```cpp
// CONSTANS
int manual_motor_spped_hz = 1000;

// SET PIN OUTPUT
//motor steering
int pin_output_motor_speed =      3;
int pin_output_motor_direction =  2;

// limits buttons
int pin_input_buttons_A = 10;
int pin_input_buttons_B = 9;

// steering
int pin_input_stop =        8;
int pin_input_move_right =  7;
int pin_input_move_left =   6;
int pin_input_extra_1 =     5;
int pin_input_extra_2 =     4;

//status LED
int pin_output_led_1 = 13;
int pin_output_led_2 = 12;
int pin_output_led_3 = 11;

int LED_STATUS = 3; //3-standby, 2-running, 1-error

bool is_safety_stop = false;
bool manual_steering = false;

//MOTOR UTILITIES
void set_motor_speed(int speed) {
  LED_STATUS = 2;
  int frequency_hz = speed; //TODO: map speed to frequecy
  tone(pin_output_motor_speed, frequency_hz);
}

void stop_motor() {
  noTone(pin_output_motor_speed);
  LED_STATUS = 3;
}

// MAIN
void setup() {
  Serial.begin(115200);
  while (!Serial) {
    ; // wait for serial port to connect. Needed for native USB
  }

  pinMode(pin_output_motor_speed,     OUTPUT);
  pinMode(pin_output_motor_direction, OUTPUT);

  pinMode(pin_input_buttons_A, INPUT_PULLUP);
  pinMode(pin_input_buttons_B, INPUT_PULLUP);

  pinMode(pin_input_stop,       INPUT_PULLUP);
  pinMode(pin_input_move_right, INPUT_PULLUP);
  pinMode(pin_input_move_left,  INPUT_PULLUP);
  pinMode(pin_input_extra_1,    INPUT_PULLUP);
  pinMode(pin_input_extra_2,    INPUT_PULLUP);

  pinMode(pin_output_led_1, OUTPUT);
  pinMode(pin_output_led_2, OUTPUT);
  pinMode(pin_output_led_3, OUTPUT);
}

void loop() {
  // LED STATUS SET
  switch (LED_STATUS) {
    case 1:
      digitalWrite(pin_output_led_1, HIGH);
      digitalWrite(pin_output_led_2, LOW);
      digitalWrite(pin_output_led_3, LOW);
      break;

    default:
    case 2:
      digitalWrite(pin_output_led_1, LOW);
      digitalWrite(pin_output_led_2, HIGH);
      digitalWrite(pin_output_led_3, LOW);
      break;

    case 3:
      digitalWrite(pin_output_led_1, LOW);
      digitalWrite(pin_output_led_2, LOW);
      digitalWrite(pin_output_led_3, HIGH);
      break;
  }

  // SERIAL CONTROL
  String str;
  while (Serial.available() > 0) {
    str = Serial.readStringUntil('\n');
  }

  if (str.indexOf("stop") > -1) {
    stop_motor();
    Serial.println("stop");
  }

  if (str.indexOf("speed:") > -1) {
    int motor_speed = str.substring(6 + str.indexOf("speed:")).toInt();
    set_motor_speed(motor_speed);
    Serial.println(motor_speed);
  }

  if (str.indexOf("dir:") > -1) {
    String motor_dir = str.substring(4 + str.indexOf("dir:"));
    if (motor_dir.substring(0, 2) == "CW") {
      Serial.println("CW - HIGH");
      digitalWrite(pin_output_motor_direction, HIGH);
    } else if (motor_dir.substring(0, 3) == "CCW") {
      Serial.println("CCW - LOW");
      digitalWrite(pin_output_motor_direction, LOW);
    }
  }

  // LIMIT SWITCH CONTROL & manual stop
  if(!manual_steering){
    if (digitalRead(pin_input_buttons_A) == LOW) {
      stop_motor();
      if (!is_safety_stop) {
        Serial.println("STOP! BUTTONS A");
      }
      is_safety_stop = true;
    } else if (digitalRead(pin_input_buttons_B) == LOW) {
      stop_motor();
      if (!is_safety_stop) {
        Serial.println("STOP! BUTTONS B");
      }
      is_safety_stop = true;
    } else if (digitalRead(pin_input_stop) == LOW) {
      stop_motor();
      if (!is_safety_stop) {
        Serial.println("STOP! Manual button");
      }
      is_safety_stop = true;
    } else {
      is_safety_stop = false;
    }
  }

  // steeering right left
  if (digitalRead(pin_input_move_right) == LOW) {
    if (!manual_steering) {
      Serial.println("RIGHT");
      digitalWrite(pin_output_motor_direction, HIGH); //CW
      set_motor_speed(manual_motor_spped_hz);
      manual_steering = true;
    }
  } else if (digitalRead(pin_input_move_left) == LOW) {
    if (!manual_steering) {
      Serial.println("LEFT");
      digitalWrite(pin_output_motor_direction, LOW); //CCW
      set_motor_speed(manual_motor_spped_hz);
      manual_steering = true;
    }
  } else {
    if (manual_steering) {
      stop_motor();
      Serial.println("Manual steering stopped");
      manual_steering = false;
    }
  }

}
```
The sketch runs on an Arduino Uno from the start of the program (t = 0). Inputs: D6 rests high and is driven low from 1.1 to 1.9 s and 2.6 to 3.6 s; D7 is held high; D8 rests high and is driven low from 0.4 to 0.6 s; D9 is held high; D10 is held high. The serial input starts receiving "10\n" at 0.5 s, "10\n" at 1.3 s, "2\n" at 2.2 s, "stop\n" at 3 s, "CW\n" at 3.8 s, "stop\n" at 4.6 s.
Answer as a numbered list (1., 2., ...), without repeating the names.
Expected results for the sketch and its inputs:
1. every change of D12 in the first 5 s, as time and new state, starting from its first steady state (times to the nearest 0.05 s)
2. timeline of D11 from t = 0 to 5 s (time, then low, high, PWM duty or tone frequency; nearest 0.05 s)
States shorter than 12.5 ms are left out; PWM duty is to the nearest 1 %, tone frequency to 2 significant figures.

1. 0 s low; 1.1 s high; 1.9 s low; 2.6 s high; 3 s low
2. 0 s high; 1.1 s low; 1.9 s high; 2.6 s low; 3 s high
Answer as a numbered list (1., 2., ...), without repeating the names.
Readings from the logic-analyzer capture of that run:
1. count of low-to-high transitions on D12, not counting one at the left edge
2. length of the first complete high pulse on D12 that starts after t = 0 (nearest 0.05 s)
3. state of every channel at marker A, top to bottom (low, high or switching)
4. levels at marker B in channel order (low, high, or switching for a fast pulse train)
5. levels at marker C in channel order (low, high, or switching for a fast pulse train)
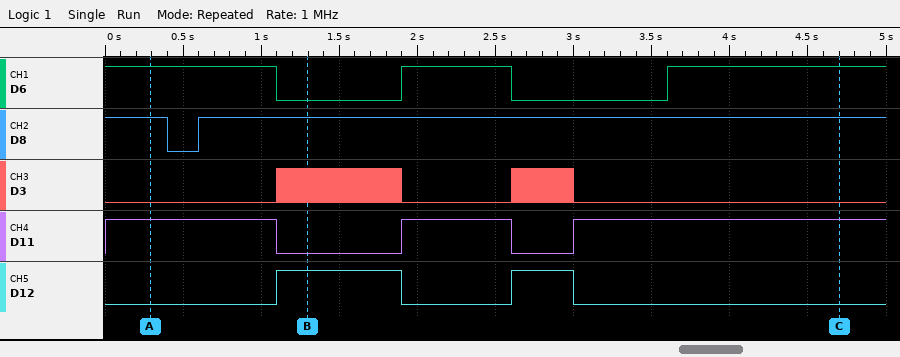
1. 2
2. 0.80 s
3. D6 high, D8 high, D3 low, D11 high, D12 low
4. D6 low, D8 high, D3 switching, D11 low, D12 high
5. D6 high, D8 high, D3 low, D11 high, D12 low
